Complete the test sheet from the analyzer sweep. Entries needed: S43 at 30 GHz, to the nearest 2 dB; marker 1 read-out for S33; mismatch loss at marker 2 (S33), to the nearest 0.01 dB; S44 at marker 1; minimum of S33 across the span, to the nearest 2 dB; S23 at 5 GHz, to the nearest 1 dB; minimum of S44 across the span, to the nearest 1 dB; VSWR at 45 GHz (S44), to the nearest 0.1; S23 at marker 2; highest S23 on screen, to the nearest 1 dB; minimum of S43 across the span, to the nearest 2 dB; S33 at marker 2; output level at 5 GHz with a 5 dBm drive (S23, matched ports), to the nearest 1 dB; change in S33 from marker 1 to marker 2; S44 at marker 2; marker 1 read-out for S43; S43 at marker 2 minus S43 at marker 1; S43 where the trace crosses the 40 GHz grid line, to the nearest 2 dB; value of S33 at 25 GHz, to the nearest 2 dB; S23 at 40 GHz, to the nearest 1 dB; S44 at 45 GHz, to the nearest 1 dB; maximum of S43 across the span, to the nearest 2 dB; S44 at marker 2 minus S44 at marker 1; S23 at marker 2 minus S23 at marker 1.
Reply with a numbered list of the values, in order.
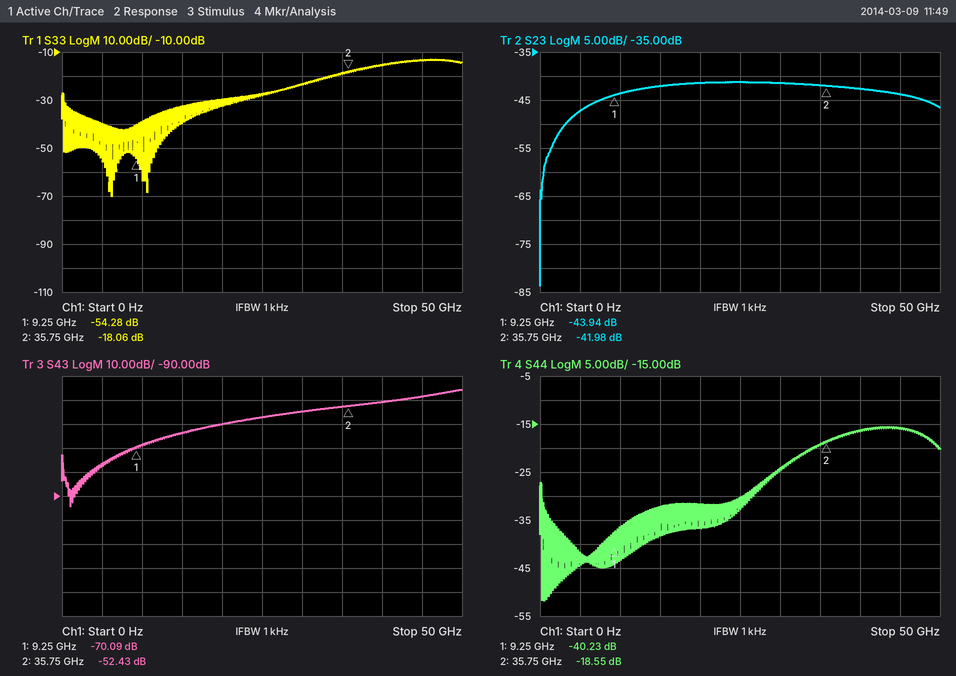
1. -54 dB
2. -54.28 dB
3. 0.07 dB
4. -40.23 dB
5. -70 dB
6. -47 dB
7. -52 dB
8. 1.4
9. -41.98 dB
10. -41 dB
11. -94 dB
12. -18.06 dB
13. -42 dBm
14. 36.22 dB
15. -18.55 dB
16. -70.09 dB
17. 17.66 dB
18. -50 dB
19. -28 dB
20. -43 dB
21. -16 dB
22. -46 dB
23. 21.68 dB
24. 1.96 dB
